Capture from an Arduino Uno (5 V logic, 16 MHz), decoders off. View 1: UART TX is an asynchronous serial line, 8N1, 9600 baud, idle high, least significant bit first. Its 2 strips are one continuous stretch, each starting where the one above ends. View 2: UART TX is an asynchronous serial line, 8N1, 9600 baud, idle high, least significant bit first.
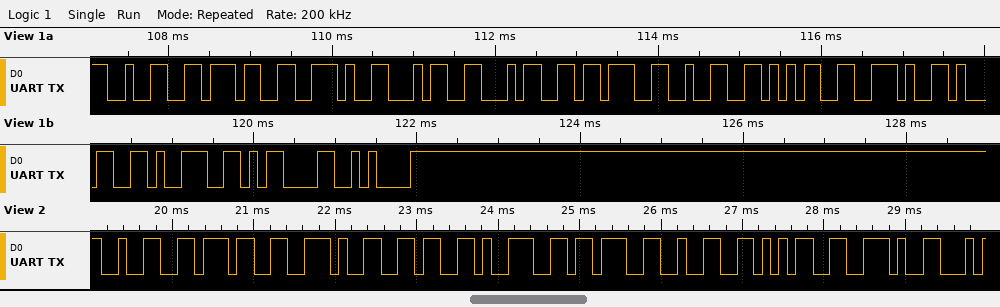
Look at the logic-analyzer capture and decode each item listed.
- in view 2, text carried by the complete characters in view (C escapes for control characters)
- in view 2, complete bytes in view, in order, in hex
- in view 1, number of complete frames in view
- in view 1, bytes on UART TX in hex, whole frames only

"27.69;25."
32 37 2E 36 39 3B 32 35 2E
13
32 37 2E 34 34 3B 32 35 2E 31 39 0D 0A
